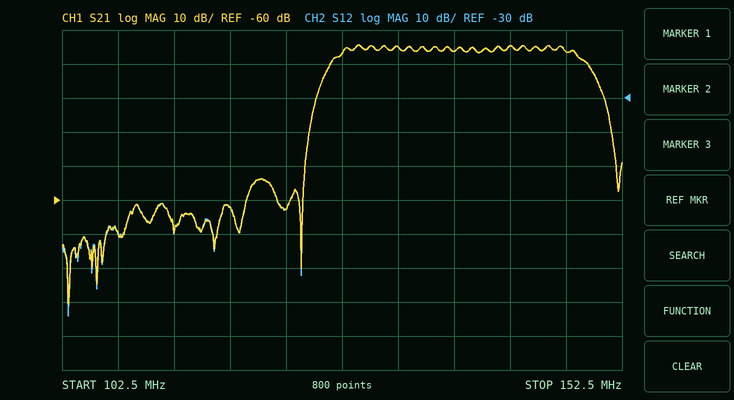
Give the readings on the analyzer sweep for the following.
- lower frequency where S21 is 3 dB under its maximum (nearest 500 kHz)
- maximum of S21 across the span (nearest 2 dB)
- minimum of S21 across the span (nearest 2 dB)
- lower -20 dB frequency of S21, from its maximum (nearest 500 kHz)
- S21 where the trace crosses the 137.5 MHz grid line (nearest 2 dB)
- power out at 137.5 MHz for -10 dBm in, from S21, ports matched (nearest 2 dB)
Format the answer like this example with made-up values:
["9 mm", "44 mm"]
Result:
["127.5 MHz", "-14 dB", "-90 dB", "125.0 MHz", "-16 dB", "-26 dBm"]
